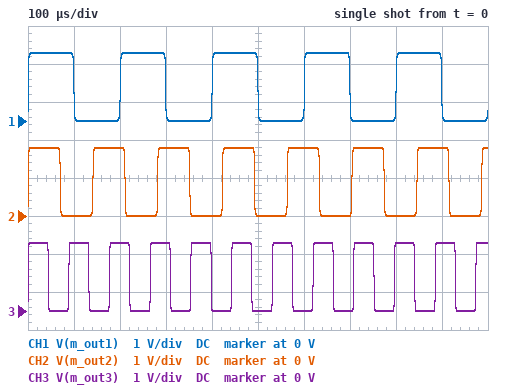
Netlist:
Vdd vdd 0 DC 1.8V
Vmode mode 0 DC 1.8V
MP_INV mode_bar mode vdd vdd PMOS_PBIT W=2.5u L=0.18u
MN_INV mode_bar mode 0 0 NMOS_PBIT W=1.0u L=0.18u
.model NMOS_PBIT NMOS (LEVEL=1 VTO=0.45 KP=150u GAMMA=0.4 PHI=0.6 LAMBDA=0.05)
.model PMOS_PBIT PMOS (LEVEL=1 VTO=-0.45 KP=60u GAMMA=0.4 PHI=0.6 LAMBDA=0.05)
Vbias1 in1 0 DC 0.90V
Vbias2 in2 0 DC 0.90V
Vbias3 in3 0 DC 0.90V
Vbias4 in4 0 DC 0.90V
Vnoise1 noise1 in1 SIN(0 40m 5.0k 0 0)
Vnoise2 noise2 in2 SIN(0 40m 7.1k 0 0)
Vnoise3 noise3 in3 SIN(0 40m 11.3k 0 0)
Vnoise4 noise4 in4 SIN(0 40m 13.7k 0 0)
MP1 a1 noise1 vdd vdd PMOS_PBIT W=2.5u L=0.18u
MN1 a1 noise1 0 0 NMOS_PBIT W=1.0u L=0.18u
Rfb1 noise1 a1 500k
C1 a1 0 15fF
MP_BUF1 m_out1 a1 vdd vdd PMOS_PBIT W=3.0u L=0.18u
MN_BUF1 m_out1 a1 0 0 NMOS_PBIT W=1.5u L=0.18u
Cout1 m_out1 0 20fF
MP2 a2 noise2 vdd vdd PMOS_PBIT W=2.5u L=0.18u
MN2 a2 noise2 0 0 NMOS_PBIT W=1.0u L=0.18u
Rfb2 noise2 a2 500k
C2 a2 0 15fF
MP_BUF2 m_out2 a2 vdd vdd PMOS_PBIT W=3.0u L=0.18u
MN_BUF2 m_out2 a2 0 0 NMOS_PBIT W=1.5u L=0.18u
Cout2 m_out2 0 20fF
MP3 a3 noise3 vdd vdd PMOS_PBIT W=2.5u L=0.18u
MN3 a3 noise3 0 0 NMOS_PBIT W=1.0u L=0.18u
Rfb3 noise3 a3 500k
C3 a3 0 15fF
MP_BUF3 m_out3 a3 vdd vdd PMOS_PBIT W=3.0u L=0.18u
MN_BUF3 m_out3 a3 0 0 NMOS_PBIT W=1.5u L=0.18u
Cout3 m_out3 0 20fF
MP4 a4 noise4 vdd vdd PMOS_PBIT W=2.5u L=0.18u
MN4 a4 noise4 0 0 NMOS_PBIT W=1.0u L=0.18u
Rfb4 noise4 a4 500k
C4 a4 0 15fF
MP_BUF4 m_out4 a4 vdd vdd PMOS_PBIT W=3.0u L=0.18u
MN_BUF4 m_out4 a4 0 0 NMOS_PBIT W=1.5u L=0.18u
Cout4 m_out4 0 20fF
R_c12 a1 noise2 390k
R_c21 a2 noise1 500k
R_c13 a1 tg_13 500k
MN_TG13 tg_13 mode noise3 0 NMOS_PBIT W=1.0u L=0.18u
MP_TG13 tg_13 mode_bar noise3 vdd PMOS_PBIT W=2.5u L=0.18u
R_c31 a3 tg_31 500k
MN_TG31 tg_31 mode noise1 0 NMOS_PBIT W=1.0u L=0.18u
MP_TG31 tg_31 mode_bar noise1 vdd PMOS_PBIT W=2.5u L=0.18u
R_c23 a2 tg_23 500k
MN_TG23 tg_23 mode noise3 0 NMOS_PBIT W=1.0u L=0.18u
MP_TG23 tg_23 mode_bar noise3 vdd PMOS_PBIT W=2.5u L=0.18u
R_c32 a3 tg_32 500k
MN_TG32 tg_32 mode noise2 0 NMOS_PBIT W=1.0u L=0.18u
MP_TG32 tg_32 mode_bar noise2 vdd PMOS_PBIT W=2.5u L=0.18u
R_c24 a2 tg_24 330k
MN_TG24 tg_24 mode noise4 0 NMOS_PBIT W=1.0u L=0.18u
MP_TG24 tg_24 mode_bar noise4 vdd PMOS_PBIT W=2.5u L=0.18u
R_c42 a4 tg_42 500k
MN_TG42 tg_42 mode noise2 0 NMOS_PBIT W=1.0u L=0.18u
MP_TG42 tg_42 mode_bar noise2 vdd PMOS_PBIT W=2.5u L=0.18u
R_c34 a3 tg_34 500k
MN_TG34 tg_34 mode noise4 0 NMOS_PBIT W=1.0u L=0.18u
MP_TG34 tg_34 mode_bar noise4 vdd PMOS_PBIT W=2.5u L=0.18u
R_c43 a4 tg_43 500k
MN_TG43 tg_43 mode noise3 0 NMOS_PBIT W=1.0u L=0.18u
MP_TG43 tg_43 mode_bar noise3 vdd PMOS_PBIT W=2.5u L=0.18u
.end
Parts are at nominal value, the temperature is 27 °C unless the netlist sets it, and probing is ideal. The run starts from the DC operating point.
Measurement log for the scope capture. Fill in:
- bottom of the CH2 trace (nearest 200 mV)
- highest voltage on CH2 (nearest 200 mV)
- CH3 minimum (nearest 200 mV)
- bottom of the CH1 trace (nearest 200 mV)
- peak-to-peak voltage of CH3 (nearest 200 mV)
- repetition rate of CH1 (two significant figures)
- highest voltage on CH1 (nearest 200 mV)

0 V
1.8 V
0 V
0 V
1.8 V
5.0 kHz
1.8 V
